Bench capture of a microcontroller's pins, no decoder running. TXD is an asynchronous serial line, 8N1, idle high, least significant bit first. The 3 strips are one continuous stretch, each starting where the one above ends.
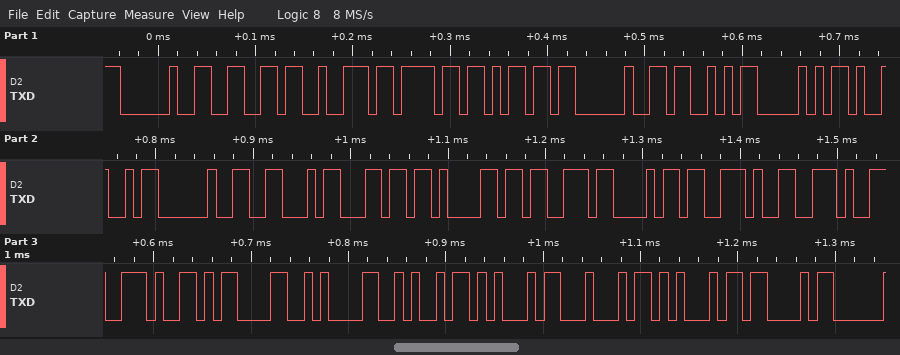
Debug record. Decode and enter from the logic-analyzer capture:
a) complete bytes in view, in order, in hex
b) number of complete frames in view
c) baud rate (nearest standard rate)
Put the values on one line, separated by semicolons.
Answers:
20 66 72 6F 6D 20 53 50 49 20 46 6C 61 73 68 2E 2E 2E 0D 0A 4A 45 44 45 43; 25; 115200 baud
